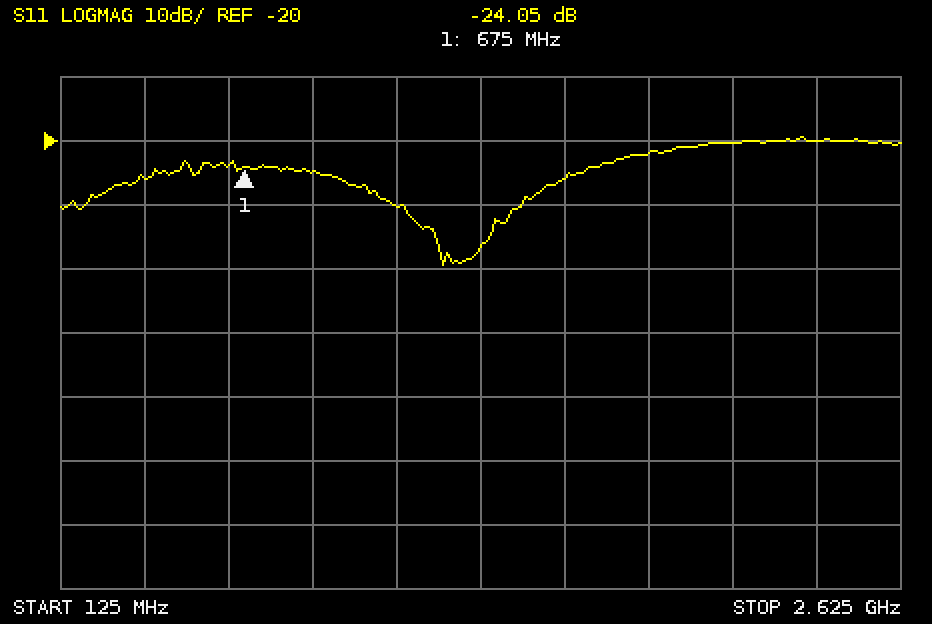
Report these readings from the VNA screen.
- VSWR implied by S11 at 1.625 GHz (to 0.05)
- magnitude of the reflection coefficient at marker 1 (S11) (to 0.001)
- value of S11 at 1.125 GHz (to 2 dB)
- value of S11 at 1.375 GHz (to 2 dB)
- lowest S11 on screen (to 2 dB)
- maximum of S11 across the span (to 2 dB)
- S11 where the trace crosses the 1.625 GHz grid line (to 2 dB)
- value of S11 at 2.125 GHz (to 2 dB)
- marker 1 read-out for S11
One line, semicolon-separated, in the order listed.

1.10; 0.063; -30 dB; -36 dB; -40 dB; -20 dB; -26 dB; -20 dB; -24.05 dB
